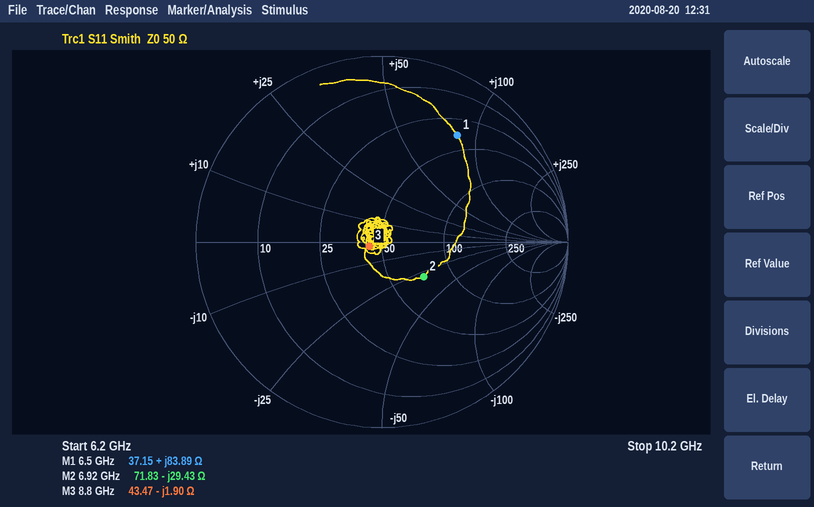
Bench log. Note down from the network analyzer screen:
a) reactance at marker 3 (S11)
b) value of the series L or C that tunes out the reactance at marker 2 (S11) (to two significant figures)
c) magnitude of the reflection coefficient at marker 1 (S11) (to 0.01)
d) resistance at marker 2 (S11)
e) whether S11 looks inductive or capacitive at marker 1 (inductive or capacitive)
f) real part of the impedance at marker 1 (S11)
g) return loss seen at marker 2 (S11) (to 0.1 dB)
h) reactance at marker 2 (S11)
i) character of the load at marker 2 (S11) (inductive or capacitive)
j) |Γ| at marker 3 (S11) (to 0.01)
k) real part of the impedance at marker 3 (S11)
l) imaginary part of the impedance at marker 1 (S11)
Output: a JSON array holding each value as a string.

["-1.90 Ω", "680 pH", "0.70", "71.83 Ω", "inductive", "37.15 Ω", "10.7 dB", "-29.43 Ω", "capacitive", "0.07", "43.47 Ω", "+83.89 Ω"]
